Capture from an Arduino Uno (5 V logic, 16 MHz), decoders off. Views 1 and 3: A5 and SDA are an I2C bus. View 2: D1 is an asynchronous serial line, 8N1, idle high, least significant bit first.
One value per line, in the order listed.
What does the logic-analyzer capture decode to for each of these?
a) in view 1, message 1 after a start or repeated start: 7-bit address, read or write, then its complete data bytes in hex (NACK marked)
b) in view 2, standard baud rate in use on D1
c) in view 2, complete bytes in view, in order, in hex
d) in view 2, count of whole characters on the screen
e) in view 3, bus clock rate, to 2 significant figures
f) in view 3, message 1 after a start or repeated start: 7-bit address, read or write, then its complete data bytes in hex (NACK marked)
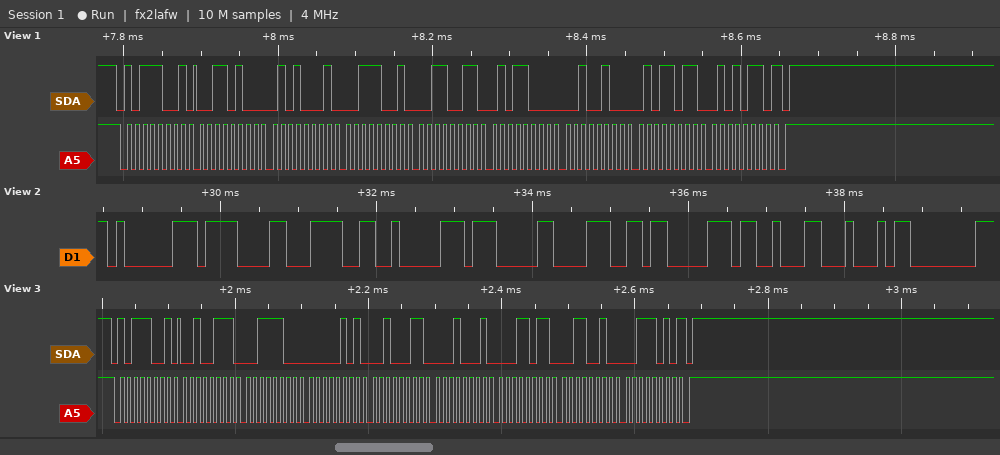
0x5C read: 34 51 39 33 58 24 5B 56 NACK
9600 baud
81 0F 3C 82 07 38 83 13 44 80
10
100 kHz
0x5C read: 27 3C 05 23 11 1B 32 3A NACK
